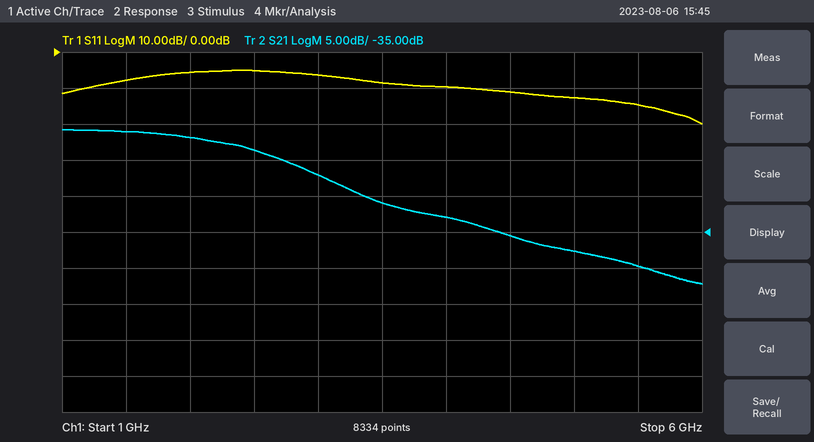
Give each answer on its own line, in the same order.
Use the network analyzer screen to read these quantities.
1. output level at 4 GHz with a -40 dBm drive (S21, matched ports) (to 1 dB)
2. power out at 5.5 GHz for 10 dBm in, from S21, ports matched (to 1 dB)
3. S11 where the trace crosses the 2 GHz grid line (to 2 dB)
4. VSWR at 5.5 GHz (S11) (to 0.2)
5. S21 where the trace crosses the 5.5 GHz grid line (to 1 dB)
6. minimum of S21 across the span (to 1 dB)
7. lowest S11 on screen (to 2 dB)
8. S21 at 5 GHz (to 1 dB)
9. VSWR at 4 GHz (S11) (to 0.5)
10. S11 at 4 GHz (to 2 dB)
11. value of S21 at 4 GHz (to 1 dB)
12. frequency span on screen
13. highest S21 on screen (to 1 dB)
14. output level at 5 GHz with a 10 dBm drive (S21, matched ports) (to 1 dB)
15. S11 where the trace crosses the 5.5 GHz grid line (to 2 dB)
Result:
-73 dBm
-30 dBm
-6 dB
1.4
-40 dB
-42 dB
-20 dB
-38 dB
2.0
-10 dB
-33 dB
5 GHz
-21 dB
-28 dBm
-14 dB
